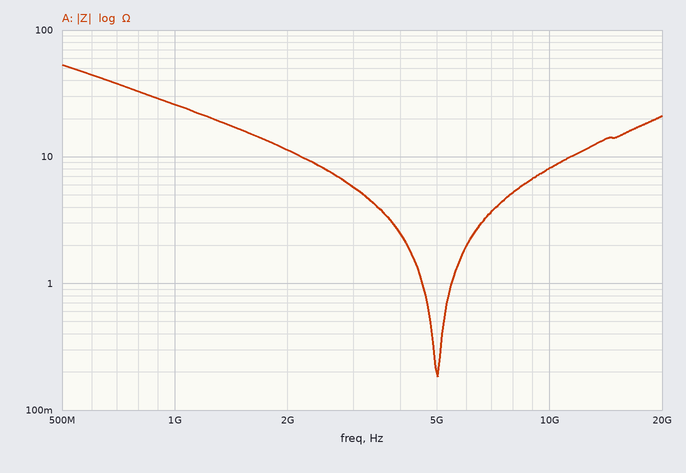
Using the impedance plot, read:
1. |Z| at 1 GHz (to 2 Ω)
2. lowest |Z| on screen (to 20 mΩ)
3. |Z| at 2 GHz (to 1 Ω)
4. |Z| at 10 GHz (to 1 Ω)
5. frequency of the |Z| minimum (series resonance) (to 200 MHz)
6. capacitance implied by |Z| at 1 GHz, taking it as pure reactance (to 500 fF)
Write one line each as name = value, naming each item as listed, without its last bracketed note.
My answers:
|Z| at 1 GHz = 26 Ω
lowest |Z| on screen = 180 mΩ
|Z| at 2 GHz = 11 Ω
|Z| at 10 GHz = 8 Ω
frequency of the |Z| minimum (series resonance) = 5.0 GHz
capacitance implied by |Z| at 1 GHz, taking it as pure reactance = 6.0 pF
